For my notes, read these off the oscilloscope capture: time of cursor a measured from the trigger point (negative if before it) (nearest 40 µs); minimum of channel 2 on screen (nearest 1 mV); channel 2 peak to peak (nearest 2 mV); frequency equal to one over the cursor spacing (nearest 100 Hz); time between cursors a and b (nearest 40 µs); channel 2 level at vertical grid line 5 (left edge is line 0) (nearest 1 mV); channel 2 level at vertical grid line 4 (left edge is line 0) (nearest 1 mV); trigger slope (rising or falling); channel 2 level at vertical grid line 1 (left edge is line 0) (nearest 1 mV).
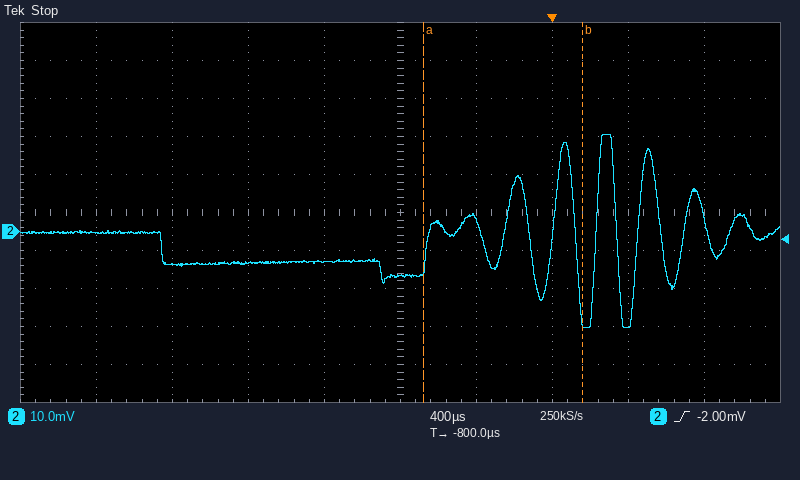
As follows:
-680 µs
-25 mV
50 mV
1.2 kHz
840 µs
-12 mV
-8 mV
rising
0 mV
